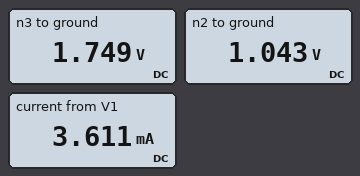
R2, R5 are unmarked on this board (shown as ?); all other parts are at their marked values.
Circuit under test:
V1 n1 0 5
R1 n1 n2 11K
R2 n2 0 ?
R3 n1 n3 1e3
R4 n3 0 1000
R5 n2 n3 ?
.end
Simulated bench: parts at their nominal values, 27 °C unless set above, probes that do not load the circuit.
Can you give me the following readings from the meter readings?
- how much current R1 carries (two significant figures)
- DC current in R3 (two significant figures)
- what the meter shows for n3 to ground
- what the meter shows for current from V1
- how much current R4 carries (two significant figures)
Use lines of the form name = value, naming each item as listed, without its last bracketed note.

how much current R1 carries = 360 µA
DC current in R3 = 3.3 mA
what the meter shows for n3 to ground = 1.749 V
what the meter shows for current from V1 = 3.611 mA
how much current R4 carries = 1.7 mA
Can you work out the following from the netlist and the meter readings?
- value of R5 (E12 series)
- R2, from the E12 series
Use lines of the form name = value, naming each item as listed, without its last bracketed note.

value of R5 = 470 Ω
R2, from the E12 series = 560 Ω
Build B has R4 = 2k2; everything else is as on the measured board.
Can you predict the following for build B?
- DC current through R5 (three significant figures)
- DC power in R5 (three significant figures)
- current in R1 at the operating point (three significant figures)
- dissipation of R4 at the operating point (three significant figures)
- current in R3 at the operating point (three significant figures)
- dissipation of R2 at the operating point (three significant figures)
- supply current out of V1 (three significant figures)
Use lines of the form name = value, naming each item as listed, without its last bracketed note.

DC current through R5 = 1.89 mA
DC power in R5 = 1.68 mW
current in R1 at the operating point = 341 µA
dissipation of R4 at the operating point = 2.08 mW
current in R3 at the operating point = 2.86 mA
dissipation of R2 at the operating point = 2.79 mW
supply current out of V1 = 3.20 mA
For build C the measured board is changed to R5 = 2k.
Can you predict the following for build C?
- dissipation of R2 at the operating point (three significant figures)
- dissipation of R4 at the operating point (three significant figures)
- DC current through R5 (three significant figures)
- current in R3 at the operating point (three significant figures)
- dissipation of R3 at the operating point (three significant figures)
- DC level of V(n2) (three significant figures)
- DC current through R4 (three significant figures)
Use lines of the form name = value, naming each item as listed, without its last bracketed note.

dissipation of R2 at the operating point = 729 µW
dissipation of R4 at the operating point = 4.53 mW
DC current through R5 = 744 µA
current in R3 at the operating point = 2.87 mA
dissipation of R3 at the operating point = 8.25 mW
DC level of V(n2) = 639 mV
DC current through R4 = 2.13 mA
